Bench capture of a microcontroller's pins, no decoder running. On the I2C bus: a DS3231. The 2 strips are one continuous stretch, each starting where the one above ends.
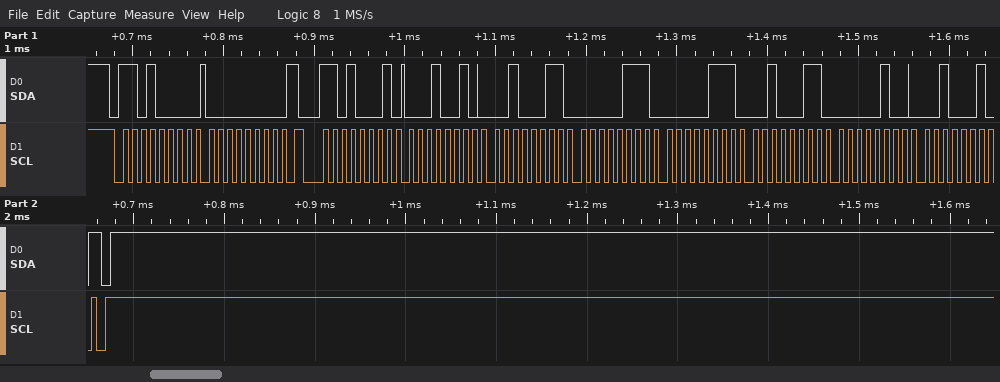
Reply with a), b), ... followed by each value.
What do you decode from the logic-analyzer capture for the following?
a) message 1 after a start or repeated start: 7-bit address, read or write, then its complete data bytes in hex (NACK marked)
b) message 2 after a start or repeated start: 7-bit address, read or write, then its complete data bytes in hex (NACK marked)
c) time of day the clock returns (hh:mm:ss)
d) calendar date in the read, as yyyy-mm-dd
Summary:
a) 0x68 write: 00
b) 0x68 read: 12 23 07 07 23 04 22 NACK
c) 07:23:12
d) 2022-04-23
